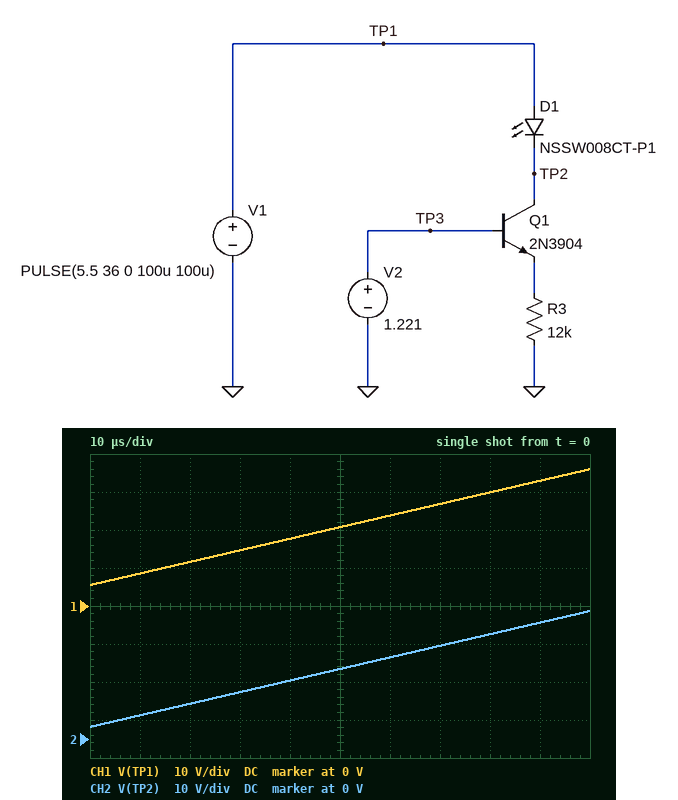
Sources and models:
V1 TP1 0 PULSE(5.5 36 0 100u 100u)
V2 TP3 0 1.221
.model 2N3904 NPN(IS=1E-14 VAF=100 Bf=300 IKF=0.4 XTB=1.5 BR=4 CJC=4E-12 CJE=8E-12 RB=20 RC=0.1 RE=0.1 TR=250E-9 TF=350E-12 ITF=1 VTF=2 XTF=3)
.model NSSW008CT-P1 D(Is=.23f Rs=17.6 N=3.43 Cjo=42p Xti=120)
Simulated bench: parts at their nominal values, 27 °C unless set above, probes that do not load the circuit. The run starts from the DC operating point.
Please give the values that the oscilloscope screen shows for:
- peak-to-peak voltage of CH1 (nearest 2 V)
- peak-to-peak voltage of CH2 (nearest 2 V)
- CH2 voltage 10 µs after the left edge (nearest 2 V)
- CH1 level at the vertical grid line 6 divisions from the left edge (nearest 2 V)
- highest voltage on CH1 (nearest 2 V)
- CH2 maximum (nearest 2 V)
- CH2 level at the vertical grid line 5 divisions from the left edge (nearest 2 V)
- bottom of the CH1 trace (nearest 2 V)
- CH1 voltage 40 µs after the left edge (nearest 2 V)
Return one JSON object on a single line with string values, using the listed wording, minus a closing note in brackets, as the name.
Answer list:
{"peak-to-peak voltage of CH1": "30 V", "peak-to-peak voltage of CH2": "30 V", "CH2 voltage 10 µs after the left edge": "6 V", "CH1 level at the vertical grid line 6 divisions from the left edge": "24 V", "highest voltage on CH1": "36 V", "CH2 maximum": "34 V", "CH2 level at the vertical grid line 5 divisions from the left edge": "18 V", "bottom of the CH1 trace": "6 V", "CH1 voltage 40 µs after the left edge": "18 V"}
